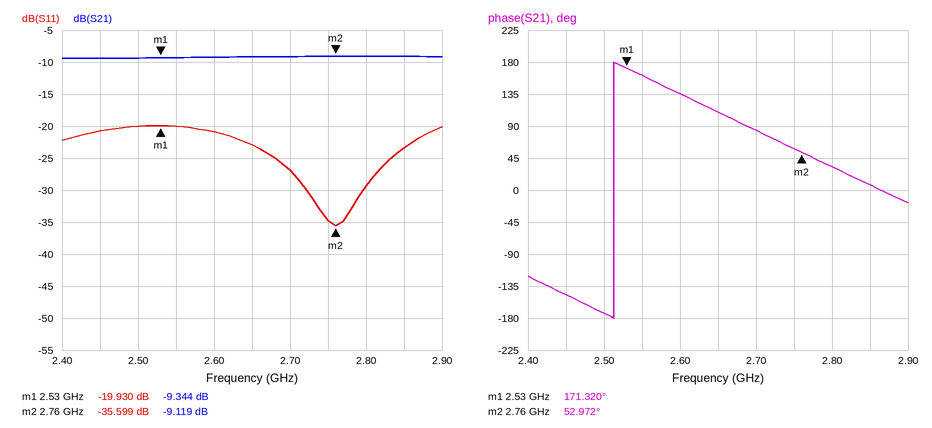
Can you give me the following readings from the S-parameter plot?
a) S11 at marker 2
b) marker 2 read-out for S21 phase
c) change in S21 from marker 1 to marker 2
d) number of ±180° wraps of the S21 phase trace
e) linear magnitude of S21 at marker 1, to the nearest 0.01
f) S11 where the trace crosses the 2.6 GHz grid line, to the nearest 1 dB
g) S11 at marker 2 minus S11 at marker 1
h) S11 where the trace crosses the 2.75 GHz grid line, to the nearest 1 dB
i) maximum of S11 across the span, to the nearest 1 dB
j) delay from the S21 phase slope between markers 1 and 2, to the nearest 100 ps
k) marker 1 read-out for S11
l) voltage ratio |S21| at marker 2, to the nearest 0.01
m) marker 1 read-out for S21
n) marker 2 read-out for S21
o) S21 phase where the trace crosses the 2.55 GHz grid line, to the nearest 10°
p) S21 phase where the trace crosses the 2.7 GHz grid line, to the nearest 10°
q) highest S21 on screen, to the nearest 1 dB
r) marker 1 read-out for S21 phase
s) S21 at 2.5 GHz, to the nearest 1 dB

-35.599 dB
52.972°
0.225 dB
1
0.34
-21 dB
-15.669 dB
-35 dB
-20 dB
1.4 ns
-19.930 dB
0.35
-9.344 dB
-9.119 dB
160°
80°
-9 dB
171.320°
-9 dB
